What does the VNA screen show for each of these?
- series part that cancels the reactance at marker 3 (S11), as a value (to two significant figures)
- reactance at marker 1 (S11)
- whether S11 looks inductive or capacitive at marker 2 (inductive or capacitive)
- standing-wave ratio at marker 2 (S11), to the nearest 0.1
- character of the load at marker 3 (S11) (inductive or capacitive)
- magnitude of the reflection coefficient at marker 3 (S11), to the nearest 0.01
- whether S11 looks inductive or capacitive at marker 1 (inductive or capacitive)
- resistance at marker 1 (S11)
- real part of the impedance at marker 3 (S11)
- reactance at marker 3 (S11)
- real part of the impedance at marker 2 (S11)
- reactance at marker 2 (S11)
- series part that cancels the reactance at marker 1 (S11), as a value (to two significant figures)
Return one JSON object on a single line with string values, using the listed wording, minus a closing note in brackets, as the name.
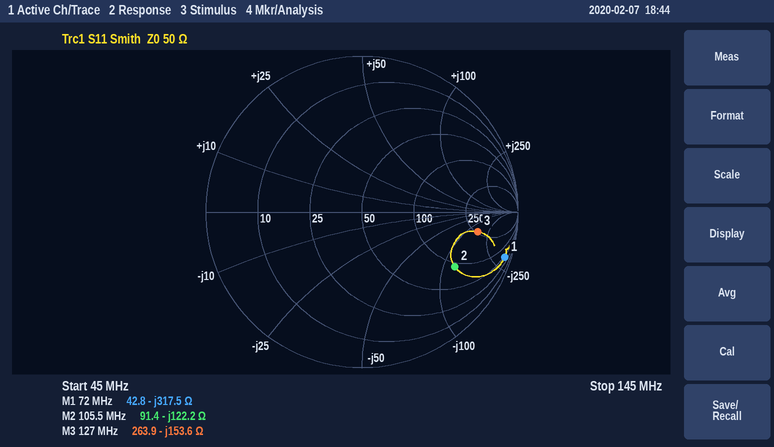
{"series part that cancels the reactance at marker 3 (S11), as a value": "190 nH", "reactance at marker 1": "-317.5 Ω", "whether S11 looks inductive or capacitive at marker 2": "capacitive", "standing-wave ratio at marker 2 (S11), to the nearest 0.1": "5.5", "character of the load at marker 3 (S11)": "capacitive", "magnitude of the reflection coefficient at marker 3 (S11), to the nearest 0.01": "0.75", "whether S11 looks inductive or capacitive at marker 1": "capacitive", "resistance at marker 1": "42.8 Ω", "real part of the impedance at marker 3": "263.9 Ω", "reactance at marker 3": "-153.6 Ω", "real part of the impedance at marker 2": "91.4 Ω", "reactance at marker 2": "-122.2 Ω", "series part that cancels the reactance at marker 1 (S11), as a value": "700 nH"}
